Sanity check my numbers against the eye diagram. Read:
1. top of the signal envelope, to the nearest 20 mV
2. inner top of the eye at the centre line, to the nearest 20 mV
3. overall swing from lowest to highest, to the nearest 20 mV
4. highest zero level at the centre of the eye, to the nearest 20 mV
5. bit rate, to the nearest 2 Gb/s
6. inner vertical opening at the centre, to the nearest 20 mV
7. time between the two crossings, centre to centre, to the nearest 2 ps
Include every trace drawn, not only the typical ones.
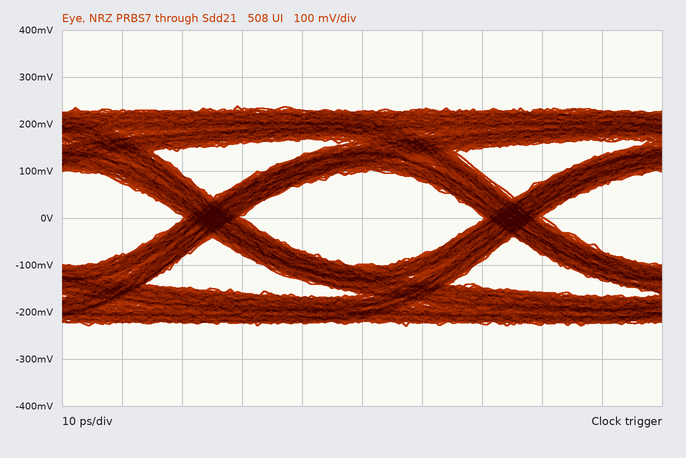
240 mV
100 mV
460 mV
-100 mV
20 Gb/s
200 mV
50 ps
